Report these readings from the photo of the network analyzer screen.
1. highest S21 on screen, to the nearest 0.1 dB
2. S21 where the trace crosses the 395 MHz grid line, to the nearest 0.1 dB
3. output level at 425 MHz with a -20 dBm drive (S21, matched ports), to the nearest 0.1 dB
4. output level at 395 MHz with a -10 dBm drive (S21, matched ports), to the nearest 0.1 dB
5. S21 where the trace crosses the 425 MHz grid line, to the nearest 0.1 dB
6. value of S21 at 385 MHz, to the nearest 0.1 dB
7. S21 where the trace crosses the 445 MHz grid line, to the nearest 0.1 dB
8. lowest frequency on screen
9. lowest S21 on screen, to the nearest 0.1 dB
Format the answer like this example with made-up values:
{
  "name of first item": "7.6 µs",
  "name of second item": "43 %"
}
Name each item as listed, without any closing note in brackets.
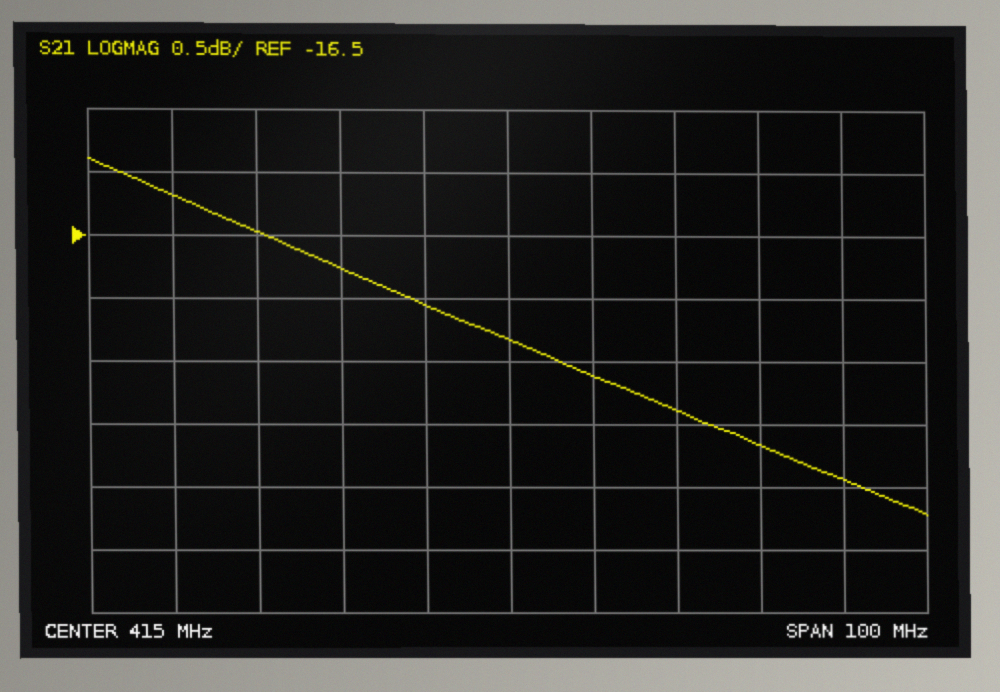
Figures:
{
  "highest S21 on screen, to the nearest 0.1 dB": "-15.9 dB",
  "S21 where the trace crosses the 395 MHz grid line, to the nearest 0.1 dB": "-16.8 dB",
  "output level at 425 MHz with a -20 dBm drive (S21, matched ports), to the nearest 0.1 dB": "-37.6 dBm",
  "output level at 395 MHz with a -10 dBm drive (S21, matched ports), to the nearest 0.1 dB": "-26.8 dBm",
  "S21 where the trace crosses the 425 MHz grid line, to the nearest 0.1 dB": "-17.6 dB",
  "value of S21 at 385 MHz, to the nearest 0.1 dB": "-16.5 dB",
  "S21 where the trace crosses the 445 MHz grid line, to the nearest 0.1 dB": "-18.2 dB",
  "lowest frequency on screen": "365 MHz",
  "lowest S21 on screen, to the nearest 0.1 dB": "-18.7 dB"
}
